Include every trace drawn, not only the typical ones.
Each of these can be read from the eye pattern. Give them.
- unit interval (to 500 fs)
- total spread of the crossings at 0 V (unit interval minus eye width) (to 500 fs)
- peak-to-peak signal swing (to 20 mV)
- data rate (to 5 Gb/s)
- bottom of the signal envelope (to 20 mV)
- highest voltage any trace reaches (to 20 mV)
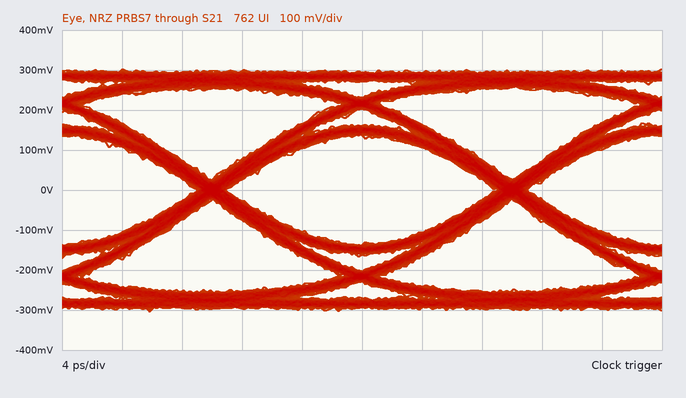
20.0 ps
2.0 ps
600 mV
50 Gb/s
-300 mV
300 mV
